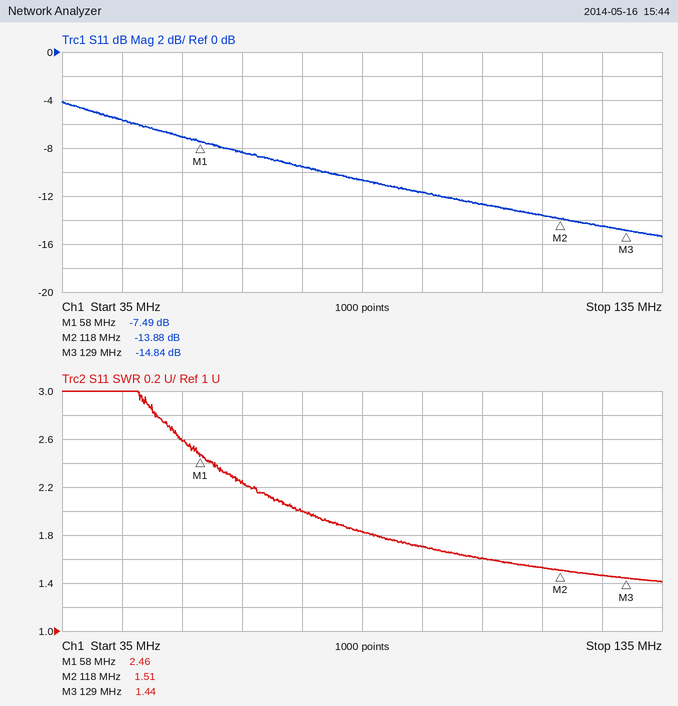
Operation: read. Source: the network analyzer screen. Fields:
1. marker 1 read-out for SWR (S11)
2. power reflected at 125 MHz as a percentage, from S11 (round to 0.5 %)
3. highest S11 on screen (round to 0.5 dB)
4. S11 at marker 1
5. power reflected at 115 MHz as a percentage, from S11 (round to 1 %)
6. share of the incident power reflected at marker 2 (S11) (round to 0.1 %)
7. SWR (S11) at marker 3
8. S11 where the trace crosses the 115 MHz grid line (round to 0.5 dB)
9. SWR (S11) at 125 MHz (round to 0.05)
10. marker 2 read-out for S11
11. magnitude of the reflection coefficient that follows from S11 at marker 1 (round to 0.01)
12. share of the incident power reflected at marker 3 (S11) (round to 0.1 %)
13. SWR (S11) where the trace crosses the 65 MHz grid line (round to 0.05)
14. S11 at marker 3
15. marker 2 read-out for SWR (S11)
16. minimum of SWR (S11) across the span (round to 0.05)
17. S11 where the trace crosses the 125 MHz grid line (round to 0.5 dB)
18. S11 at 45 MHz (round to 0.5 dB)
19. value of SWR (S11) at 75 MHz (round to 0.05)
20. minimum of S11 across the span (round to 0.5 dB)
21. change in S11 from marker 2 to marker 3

2.46
3.5 %
-4.0 dB
-7.49 dB
4 %
4.1 %
1.44
-13.5 dB
1.45
-13.88 dB
0.42
3.3 %
2.25
-14.84 dB
1.51
1.40
-14.5 dB
-5.5 dB
2.00
-15.5 dB
-0.96 dB
